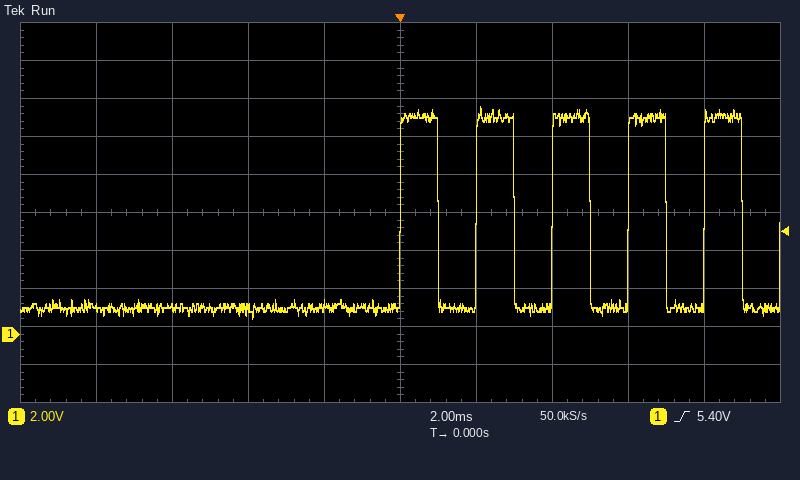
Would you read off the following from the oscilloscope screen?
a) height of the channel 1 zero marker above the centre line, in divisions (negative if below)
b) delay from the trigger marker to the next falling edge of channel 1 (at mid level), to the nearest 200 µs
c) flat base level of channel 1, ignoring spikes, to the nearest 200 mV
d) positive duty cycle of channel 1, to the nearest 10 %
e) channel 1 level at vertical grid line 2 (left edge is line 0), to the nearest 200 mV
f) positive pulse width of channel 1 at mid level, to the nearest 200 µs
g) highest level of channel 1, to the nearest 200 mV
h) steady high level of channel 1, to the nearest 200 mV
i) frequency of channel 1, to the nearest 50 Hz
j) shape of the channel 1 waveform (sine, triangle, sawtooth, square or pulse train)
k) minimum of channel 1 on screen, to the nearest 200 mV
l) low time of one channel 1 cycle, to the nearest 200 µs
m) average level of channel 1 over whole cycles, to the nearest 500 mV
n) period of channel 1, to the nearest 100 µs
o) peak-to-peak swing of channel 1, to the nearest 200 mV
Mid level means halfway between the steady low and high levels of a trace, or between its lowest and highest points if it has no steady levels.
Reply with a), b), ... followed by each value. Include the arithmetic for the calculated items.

a) -3.2 div
b) 1.0 ms
c) 1.4 V
d) 1.0 ms / 2.0 ms ≈ 50 %
e) 1.4 V
f) 1.0 ms
g) 12.0 V
h) 11.4 V
i) 1 / 2.0 ms ≈ 500 Hz
j) square
k) 800 mV
l) 1.0 ms
m) 1.4 V + 0.5 × (11.4 V − (1.4 V)) ≈ 6.40 V, so 6.5 V to the nearest 500 mV
n) 2.0 ms
o) 12.0 V − (800 mV) = 11.2 V
